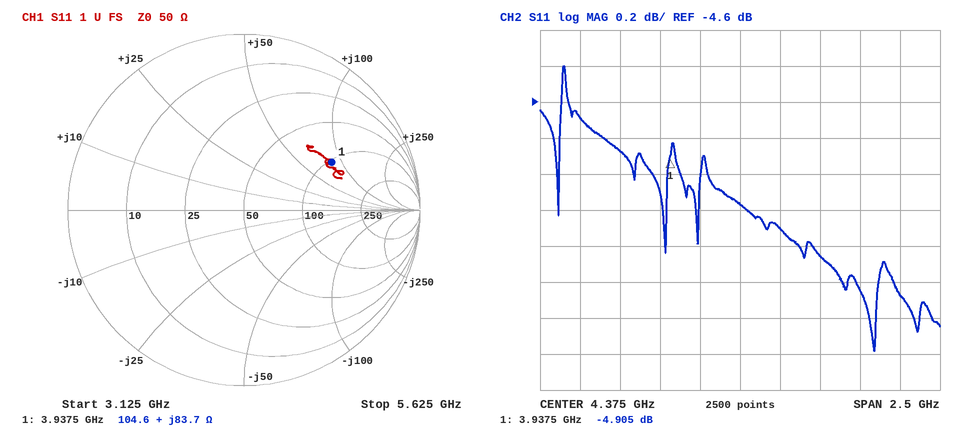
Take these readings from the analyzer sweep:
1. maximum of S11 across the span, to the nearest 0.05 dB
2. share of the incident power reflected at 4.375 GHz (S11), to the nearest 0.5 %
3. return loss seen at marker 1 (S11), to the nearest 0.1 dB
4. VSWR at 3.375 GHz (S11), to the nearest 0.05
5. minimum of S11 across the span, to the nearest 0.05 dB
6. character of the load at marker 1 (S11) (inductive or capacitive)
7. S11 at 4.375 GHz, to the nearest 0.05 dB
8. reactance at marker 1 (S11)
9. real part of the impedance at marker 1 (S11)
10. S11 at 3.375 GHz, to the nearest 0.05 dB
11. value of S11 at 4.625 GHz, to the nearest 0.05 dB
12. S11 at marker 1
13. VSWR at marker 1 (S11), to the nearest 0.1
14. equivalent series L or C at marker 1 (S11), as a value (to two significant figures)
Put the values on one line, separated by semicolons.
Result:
-4.40 dB; 30.5 %; 4.9 dB; 3.80; -6.00 dB; inductive; -5.15 dB; +83.7 Ω; 104.6 Ω; -4.70 dB; -5.30 dB; -4.905 dB; 3.6; 3.4 nH
